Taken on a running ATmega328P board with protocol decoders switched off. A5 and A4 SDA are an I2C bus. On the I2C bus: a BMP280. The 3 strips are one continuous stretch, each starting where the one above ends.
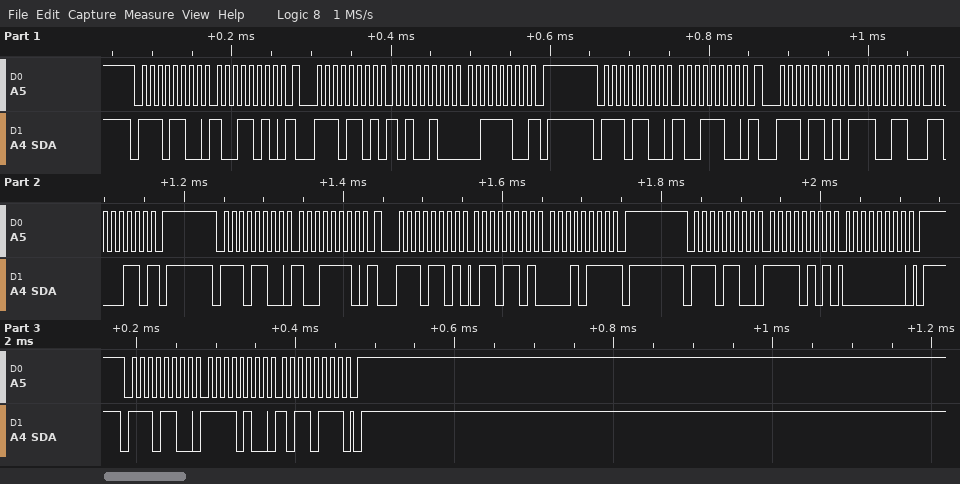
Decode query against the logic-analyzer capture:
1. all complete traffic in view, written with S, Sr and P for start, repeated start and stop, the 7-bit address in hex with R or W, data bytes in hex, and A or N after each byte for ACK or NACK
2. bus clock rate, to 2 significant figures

S 76W A 9A A Sr 76R A A4 A 3C N P S 76W A 9C A Sr 76R A E6 A C6 N P S 76W A 9E A Sr 76R A 6D A 17 N P S 76W A F5 A 00 A P S 76W A F4 A B7 A P
100 kHz
